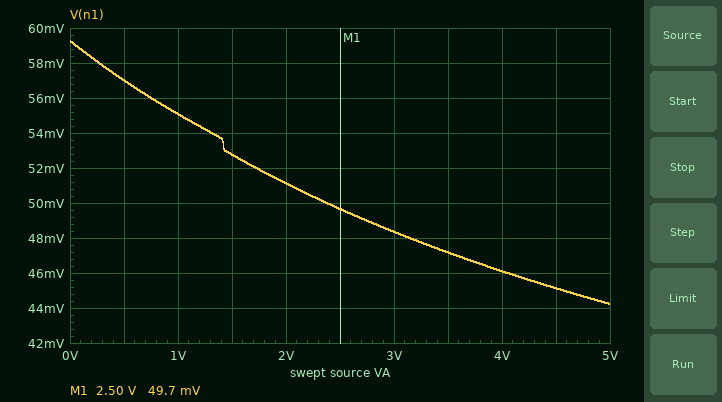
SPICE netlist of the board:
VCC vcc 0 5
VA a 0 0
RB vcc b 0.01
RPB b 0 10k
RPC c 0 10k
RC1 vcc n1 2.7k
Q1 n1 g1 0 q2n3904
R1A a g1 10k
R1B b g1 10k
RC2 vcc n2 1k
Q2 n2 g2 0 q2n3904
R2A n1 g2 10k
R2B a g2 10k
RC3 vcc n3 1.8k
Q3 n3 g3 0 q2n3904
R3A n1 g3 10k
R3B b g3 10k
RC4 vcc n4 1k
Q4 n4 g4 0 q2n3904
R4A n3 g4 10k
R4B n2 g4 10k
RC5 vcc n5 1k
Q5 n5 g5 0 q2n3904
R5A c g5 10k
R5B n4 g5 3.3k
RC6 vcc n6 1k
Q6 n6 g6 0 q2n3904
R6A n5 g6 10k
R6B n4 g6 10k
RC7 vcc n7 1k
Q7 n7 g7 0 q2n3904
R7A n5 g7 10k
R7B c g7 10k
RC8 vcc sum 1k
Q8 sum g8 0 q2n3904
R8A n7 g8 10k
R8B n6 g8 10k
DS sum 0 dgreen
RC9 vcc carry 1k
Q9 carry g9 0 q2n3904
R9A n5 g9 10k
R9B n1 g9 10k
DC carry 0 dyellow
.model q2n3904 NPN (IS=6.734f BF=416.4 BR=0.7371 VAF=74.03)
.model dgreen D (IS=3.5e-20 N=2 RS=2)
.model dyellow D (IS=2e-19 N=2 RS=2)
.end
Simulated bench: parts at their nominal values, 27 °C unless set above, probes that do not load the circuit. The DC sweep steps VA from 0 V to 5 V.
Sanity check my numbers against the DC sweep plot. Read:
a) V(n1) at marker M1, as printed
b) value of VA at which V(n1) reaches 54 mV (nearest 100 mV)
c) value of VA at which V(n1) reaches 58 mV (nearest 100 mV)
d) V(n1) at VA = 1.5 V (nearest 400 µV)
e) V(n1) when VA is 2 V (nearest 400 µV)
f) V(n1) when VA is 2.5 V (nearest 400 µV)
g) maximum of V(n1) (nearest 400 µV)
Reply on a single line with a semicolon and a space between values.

49.7 mV; 1.3 V; 300 mV; 52.8 mV; 51.2 mV; 49.6 mV; 59.2 mV
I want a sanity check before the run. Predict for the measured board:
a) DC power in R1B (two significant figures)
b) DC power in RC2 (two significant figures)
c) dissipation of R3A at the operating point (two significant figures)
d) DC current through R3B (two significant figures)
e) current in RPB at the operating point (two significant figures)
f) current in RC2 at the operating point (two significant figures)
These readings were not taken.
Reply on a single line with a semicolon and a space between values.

1.9 mW; 150 µW; 41 µW; 430 µA; 500 µA; 390 µA
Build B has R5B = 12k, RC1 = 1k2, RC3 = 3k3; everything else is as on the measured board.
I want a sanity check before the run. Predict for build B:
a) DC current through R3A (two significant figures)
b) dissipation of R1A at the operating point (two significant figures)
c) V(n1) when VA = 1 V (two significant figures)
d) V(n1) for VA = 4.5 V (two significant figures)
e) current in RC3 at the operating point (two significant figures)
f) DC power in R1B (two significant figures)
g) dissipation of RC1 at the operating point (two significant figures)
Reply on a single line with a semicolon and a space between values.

61 µA; 50 µW; 71 mV; 59 mV; 1.5 mA; 1.8 mW; 20 mW
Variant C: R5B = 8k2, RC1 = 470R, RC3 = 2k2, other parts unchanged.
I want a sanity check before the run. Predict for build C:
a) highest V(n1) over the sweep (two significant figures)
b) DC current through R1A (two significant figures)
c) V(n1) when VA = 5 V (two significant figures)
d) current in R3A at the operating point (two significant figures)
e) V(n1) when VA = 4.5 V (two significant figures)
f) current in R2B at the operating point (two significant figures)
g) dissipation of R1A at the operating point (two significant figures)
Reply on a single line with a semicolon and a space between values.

99 mV; 73 µA; 77 mV; 59 µA; 79 mV; 5.0 µA; 53 µW
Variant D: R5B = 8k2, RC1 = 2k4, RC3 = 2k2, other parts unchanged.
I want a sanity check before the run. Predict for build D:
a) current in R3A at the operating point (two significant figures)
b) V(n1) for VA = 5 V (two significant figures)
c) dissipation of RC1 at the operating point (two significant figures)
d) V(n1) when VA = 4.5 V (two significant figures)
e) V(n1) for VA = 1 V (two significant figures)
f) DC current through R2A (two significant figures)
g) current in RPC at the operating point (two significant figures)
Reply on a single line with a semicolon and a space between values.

63 µA; 46 mV; 10 mW; 47 mV; 57 mV; 3.1 µA; 30 µA
